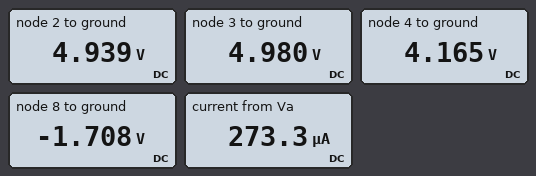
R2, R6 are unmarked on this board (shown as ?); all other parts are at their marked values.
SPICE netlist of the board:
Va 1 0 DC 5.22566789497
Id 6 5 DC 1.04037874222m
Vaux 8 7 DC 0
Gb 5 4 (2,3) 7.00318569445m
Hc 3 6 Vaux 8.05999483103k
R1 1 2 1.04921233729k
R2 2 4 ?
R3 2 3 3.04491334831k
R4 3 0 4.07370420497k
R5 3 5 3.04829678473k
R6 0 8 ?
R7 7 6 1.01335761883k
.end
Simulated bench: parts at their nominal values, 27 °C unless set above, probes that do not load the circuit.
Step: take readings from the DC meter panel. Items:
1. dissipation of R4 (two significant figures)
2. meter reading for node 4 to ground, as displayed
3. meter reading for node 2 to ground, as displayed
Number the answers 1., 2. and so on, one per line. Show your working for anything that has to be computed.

1. (4.98 V)^2 / 4.074 kΩ = 6.1 mW
2. 4.165 V
3. 4.939 V
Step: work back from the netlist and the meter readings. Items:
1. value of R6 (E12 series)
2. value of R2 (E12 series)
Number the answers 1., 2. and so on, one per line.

1. 1.8 kΩ
2. 2.7 kΩ
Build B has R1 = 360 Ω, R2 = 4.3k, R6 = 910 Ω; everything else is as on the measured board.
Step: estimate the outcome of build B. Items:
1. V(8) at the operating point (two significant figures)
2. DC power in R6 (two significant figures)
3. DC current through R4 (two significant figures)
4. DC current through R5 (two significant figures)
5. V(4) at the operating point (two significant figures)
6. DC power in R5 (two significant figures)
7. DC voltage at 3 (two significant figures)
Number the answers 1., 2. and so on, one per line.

1. -760 mV
2. 640 µW
3. 1.3 mA
4. 1.5 mA
5. 3.2 V
6. 6.7 mW
7. 5.1 V
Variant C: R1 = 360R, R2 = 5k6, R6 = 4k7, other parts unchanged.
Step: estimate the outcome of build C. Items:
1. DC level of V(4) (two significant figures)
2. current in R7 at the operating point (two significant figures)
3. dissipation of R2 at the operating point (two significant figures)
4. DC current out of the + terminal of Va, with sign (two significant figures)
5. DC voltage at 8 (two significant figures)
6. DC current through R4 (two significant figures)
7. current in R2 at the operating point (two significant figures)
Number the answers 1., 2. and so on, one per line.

1. 11 V
2. 2.3 mA
3. 5.9 mW
4. -980 µA
5. -11 V
6. 1.3 mA
7. 1.0 mA
